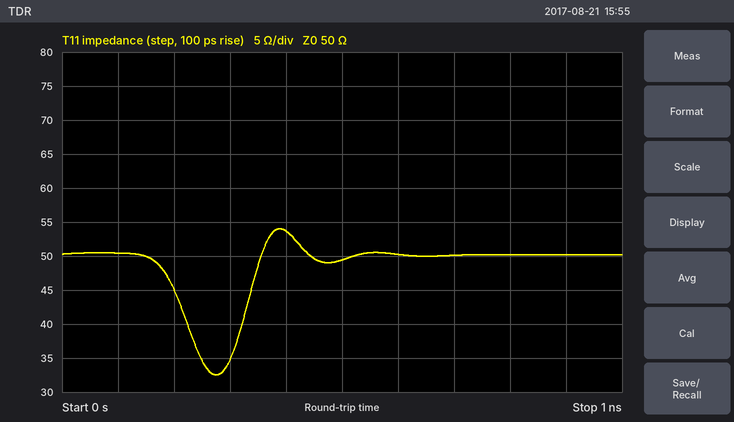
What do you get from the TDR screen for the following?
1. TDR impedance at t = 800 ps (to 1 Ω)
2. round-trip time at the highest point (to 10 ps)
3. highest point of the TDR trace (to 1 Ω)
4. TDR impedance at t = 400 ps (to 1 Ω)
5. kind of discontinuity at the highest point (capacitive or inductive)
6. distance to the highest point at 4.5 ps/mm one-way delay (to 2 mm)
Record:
50 Ω
390 ps
54 Ω
54 Ω
inductive
44 mm
